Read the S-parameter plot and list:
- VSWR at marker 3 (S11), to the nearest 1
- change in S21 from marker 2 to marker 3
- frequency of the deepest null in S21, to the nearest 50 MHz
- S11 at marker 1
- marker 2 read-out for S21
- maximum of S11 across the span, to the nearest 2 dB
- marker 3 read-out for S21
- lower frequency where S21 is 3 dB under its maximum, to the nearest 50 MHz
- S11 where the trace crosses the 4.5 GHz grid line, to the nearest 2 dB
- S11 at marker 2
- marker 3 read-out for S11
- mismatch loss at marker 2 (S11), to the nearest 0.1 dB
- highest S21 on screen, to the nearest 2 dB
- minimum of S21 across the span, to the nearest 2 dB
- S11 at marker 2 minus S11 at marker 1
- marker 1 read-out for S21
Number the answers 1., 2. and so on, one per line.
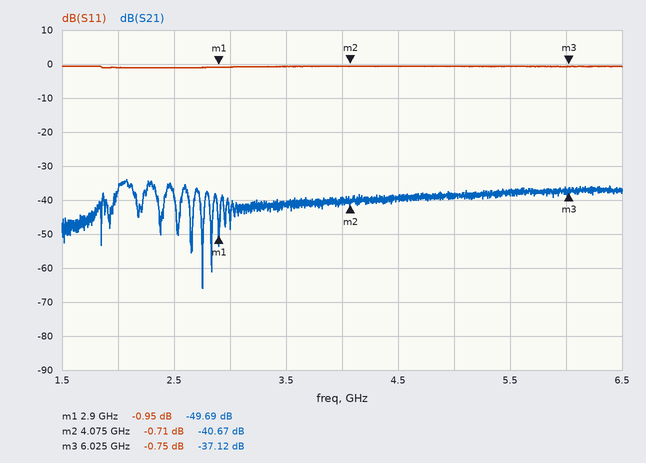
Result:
1. 23
2. 3.55 dB
3. 2.75 GHz
4. -0.95 dB
5. -40.67 dB
6. 0 dB
7. -37.12 dB
8. 2.00 GHz
9. 0 dB
10. -0.71 dB
11. -0.75 dB
12. 8.2 dB
13. -34 dB
14. -66 dB
15. 0.24 dB
16. -49.69 dB
